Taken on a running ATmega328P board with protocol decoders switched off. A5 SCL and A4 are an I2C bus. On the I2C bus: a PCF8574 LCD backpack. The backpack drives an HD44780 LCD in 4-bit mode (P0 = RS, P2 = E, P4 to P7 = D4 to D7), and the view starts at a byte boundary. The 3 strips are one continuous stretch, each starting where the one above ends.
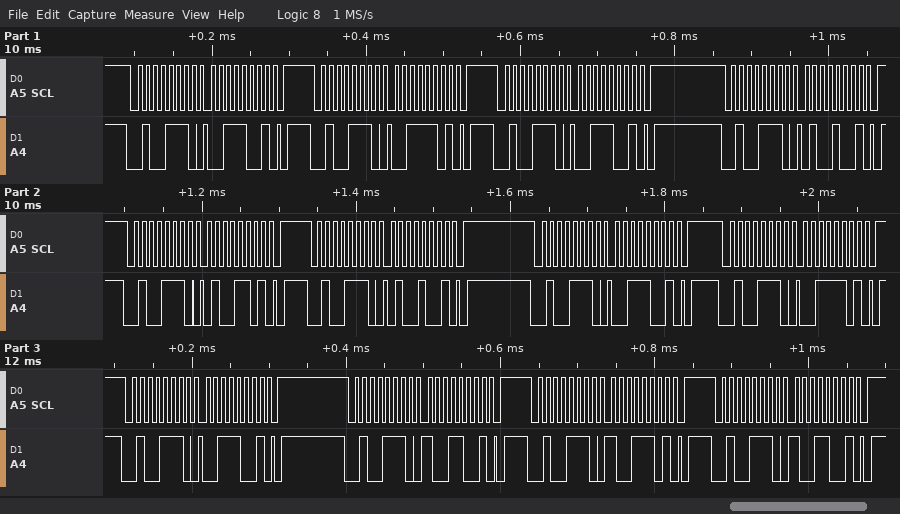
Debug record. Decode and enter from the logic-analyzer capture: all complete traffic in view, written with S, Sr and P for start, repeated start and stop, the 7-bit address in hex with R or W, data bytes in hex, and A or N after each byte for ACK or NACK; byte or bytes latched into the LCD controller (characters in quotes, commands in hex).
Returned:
S 27W A 39 A P S 27W A 3D A P S 27W A 39 A P S 27W A 49 A P S 27W A 4D A P S 27W A 49 A P S 27W A 39 A P S 27W A 3D A P S 27W A 39 A P S 27W A 99 A P S 27W A 9D A P S 27W A 99 A P
'4' '9'
